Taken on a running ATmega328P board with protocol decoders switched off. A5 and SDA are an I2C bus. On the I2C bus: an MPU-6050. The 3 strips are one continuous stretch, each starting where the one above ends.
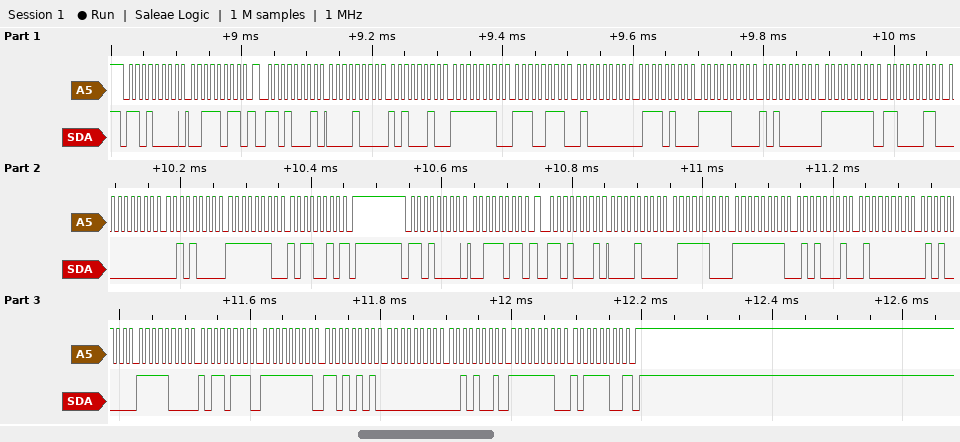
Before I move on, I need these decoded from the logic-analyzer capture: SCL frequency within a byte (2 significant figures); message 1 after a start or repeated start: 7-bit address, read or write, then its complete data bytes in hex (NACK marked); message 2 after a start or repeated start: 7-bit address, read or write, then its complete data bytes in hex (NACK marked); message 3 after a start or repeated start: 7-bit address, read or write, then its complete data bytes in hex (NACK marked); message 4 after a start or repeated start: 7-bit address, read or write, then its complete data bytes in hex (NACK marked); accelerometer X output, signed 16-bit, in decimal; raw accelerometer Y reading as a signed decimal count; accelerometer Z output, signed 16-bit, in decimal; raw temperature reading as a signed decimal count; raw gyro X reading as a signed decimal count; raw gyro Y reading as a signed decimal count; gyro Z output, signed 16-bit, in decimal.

100 kHz
0x68 write: 3B
0x68 read: 08 A2 FE E7 40 74 F8 A0 FF C3 00 28 FE B2 NACK
0x68 write: 3B
0x68 read: 08 7C FF 51 40 50 F8 B7 FF D5 00 29 FE BC NACK
2210
-281
16500
-1888
-61
40
-334
